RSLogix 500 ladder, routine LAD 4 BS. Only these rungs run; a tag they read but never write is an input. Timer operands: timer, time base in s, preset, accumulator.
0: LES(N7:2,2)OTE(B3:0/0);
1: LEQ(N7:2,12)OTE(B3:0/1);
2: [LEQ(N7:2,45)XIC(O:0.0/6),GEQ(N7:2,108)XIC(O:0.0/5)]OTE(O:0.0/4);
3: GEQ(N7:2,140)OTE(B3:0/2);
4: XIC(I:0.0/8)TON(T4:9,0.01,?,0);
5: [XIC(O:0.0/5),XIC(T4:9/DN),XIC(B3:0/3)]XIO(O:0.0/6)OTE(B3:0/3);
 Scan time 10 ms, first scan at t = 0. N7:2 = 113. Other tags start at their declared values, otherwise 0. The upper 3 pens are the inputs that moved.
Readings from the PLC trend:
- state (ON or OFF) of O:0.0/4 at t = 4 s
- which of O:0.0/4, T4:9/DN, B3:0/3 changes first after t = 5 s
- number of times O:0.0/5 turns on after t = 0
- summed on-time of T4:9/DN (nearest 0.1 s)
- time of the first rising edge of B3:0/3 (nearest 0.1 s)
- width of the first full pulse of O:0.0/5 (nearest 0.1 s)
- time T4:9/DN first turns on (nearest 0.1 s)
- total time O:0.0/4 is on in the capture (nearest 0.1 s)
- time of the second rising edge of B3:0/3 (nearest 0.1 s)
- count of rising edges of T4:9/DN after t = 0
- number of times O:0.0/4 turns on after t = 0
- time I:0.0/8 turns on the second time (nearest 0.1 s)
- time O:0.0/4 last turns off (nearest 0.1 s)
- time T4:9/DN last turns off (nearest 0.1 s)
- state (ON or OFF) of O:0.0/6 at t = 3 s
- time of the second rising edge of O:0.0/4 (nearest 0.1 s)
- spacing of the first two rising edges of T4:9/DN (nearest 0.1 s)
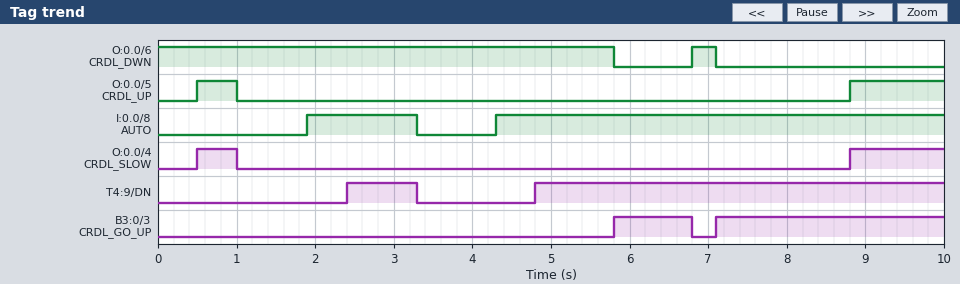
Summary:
OFF
B3:0/3
2
6.1 s
5.8 s
0.5 s
2.4 s
1.7 s
7.1 s
2
2
4.3 s
1.0 s
3.3 s
ON
8.8 s
2.4 s
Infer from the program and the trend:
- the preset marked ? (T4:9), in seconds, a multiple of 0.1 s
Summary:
0.5 s
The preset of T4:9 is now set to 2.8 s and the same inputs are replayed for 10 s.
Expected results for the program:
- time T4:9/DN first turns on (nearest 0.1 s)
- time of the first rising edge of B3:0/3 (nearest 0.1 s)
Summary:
7.1 s
7.1 s
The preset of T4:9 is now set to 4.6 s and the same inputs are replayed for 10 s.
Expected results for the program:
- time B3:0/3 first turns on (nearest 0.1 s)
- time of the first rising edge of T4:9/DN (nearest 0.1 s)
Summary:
8.8 s
8.9 s
